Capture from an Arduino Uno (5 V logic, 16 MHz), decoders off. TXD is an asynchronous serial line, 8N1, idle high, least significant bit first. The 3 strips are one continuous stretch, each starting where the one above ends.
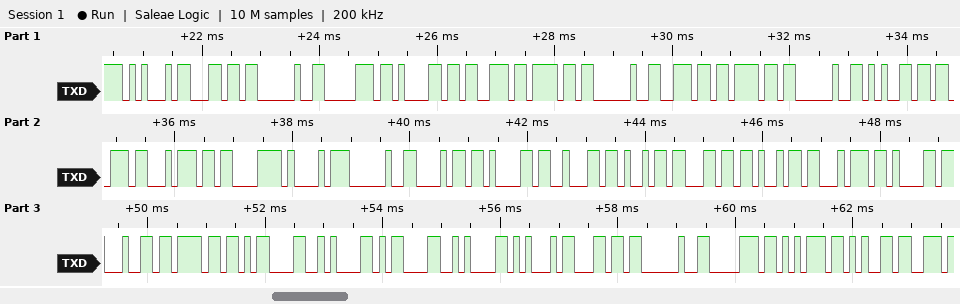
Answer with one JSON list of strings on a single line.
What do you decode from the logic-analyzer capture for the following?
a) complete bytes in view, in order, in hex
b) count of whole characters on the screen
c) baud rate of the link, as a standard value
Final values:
["45 6C 20 70 61 73 6F 20 6E 6F 20 65 73 74 C3 A1 20 68 61 62 69 6C 69 74 61 64 6F 0D 0A 0D 0A 45 6C 20 70 75 65", "37", "9600 baud"]
